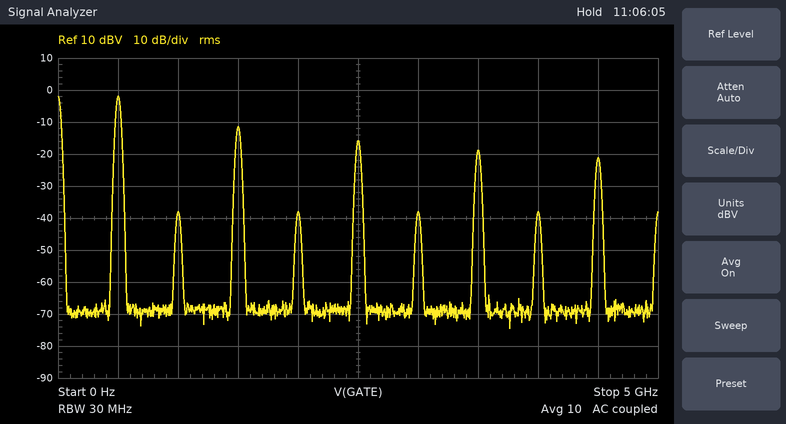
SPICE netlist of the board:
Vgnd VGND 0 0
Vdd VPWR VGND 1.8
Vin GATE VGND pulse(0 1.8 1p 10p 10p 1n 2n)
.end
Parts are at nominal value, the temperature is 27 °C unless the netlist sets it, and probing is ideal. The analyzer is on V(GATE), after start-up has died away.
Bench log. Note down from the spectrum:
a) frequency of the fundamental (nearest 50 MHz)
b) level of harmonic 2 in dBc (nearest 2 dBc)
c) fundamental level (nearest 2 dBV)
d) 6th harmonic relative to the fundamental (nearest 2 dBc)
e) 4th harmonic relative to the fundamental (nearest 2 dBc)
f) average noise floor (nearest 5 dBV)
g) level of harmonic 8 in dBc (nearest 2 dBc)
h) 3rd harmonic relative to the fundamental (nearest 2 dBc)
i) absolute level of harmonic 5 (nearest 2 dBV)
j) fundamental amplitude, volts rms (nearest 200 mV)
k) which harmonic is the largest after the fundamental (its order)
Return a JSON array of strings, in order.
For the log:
["500 MHz", "-36 dBc", "-2 dBV", "-36 dBc", "-36 dBc", "-70 dBV", "-36 dBc", "-10 dBc", "-16 dBV", "800 mV", "3"]
